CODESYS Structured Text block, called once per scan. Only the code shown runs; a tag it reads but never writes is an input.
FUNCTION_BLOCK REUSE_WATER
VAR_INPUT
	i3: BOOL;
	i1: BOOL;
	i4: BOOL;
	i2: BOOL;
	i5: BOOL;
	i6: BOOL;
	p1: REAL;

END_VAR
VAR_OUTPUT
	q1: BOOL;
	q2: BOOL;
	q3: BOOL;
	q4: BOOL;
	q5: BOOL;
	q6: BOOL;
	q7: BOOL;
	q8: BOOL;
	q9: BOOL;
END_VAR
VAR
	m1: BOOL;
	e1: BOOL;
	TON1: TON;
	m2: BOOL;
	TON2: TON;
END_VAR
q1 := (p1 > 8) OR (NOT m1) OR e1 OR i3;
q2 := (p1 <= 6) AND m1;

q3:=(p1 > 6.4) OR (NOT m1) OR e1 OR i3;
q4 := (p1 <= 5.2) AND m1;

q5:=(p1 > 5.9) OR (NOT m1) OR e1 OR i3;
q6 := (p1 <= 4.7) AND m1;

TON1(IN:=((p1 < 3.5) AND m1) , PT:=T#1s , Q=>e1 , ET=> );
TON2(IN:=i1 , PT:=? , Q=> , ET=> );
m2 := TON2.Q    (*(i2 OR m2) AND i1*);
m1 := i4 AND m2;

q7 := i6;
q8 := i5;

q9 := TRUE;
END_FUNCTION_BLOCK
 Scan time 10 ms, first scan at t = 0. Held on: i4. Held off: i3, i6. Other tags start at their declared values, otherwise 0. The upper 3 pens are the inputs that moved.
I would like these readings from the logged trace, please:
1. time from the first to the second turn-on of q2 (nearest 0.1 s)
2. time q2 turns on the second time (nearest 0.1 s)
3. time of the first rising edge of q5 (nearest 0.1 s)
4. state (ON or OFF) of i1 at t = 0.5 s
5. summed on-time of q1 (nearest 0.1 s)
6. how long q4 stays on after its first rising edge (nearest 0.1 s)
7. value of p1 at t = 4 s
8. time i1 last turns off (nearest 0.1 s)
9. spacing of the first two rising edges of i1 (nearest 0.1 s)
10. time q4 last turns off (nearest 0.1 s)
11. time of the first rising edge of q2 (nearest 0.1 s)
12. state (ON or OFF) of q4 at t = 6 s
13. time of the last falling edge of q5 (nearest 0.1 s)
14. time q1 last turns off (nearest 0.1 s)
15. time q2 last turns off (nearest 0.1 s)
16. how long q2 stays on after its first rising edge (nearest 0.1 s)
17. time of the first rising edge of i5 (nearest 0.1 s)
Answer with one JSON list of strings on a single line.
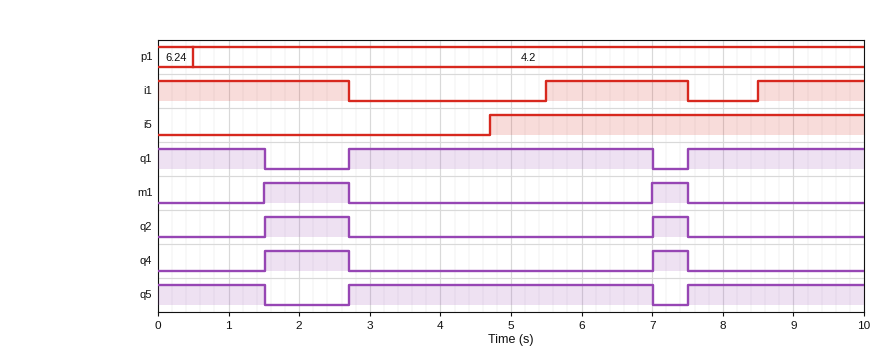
["5.5 s", "7.0 s", "2.7 s", "ON", "8.3 s", "1.2 s", "4.2", "7.5 s", "3.0 s", "7.5 s", "1.5 s", "OFF", "7.0 s", "7.0 s", "7.5 s", "1.2 s", "4.7 s"]
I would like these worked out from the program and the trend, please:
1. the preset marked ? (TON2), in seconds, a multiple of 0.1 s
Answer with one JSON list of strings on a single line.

["1.5 s"]
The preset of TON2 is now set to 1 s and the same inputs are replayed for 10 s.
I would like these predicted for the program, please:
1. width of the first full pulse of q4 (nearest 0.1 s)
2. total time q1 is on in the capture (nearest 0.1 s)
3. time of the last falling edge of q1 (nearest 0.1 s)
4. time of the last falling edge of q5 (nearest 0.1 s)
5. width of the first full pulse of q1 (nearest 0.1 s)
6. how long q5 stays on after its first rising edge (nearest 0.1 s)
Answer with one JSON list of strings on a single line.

["1.7 s", "6.8 s", "9.5 s", "9.5 s", "3.8 s", "3.8 s"]
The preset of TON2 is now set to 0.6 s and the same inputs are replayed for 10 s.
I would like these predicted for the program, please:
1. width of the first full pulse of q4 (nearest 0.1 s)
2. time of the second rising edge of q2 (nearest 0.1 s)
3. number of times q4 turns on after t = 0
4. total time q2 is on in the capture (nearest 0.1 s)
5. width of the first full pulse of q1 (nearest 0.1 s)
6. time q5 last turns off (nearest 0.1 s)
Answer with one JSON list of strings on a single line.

["2.1 s", "6.1 s", "3", "4.4 s", "3.4 s", "9.1 s"]
